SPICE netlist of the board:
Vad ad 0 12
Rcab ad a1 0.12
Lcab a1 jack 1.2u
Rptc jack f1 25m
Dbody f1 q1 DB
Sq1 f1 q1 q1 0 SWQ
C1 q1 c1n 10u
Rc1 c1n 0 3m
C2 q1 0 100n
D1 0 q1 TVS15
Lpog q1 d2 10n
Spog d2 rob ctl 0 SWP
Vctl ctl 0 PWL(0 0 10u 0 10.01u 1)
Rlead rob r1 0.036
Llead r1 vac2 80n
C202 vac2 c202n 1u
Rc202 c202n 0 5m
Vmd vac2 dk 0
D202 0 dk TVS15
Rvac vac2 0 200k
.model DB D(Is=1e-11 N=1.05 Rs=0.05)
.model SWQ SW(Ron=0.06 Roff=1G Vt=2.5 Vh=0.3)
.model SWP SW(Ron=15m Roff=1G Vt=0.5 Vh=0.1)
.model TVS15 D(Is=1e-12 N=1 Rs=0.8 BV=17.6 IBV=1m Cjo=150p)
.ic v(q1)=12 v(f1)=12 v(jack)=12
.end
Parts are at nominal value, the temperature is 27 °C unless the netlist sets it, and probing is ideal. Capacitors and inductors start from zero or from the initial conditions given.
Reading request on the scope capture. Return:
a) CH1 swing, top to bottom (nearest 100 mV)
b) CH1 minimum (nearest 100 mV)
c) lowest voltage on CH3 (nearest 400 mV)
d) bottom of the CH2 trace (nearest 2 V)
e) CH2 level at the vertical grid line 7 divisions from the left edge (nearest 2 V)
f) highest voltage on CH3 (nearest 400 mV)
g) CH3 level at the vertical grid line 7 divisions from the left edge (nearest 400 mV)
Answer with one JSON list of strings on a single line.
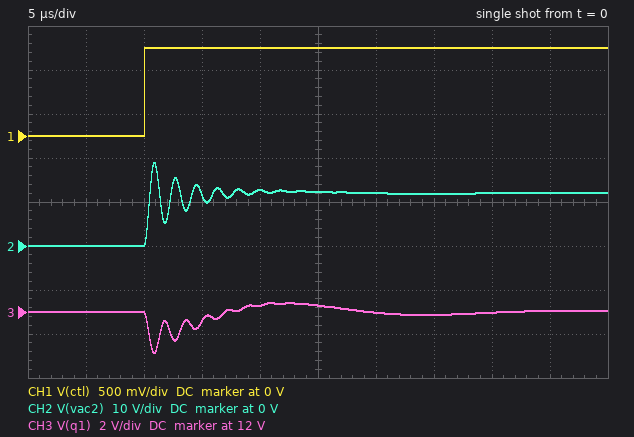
["1.0 V", "0 V", "10.0 V", "0 V", "12 V", "12.4 V", "12.0 V"]
